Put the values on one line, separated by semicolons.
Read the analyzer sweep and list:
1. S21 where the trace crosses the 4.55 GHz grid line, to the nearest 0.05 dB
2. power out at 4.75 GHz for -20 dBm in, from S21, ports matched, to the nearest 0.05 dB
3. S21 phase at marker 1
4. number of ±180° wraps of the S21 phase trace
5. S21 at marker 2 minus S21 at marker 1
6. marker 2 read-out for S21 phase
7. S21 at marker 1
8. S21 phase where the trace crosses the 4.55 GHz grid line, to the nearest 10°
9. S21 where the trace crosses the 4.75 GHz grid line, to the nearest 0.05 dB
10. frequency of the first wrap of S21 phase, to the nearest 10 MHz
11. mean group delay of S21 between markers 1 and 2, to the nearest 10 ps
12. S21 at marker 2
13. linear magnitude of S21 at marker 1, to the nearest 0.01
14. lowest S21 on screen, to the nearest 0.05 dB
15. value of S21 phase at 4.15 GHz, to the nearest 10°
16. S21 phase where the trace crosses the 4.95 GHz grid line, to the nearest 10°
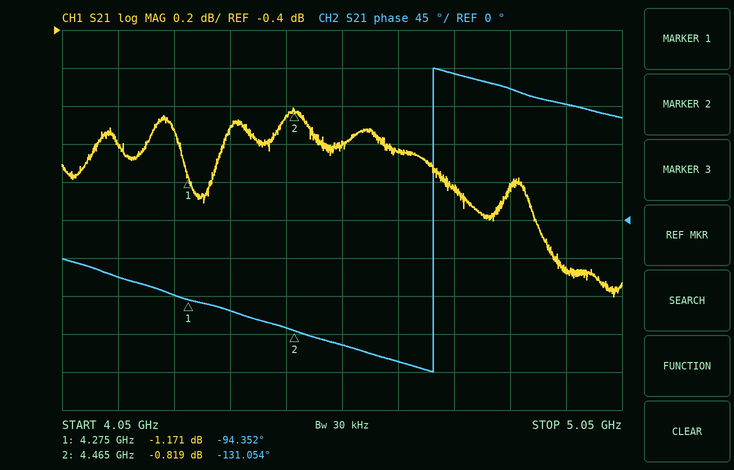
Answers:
-1.00 dB; -21.25 dBm; -94.352°; 1; 0.352 dB; -131.054°; -1.171 dB; -150°; -1.25 dB; 4.71 GHz; 540 ps; -0.819 dB; 0.87; -1.80 dB; -70°; 140°
